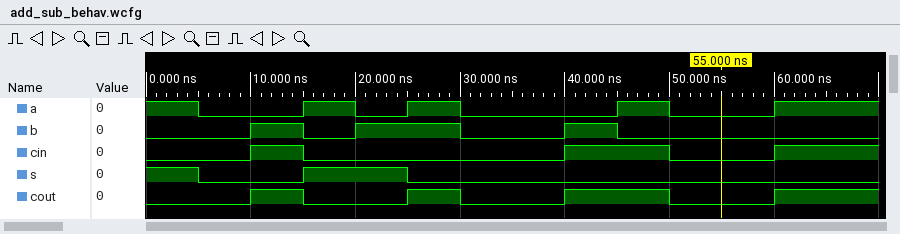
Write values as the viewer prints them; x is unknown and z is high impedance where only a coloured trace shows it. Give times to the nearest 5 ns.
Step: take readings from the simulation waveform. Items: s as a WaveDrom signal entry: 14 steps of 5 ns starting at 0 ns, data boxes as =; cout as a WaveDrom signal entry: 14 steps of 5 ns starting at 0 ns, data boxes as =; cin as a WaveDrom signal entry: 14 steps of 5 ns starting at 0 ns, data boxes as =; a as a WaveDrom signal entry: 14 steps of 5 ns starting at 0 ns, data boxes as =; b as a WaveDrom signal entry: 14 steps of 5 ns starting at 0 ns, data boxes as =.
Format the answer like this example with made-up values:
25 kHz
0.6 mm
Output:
{name: 's', wave: '10.1.0........'}
{name: 'cout', wave: '0.10.10.1.0.1.'}
{name: 'cin', wave: '0.10....1.0.1.'}
{name: 'a', wave: '10.1010..10.1.'}
{name: 'b', wave: '0.101.0.10....'}
